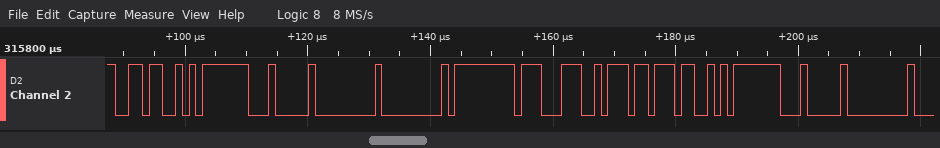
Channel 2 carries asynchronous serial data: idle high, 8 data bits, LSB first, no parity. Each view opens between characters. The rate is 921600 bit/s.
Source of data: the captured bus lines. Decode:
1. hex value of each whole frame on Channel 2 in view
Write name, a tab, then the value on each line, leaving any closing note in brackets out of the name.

hex value of each whole frame on Channel 2 in view	36, FD, 04, 00, 00, FF, C7, BA, 37, FD, 04, 00
